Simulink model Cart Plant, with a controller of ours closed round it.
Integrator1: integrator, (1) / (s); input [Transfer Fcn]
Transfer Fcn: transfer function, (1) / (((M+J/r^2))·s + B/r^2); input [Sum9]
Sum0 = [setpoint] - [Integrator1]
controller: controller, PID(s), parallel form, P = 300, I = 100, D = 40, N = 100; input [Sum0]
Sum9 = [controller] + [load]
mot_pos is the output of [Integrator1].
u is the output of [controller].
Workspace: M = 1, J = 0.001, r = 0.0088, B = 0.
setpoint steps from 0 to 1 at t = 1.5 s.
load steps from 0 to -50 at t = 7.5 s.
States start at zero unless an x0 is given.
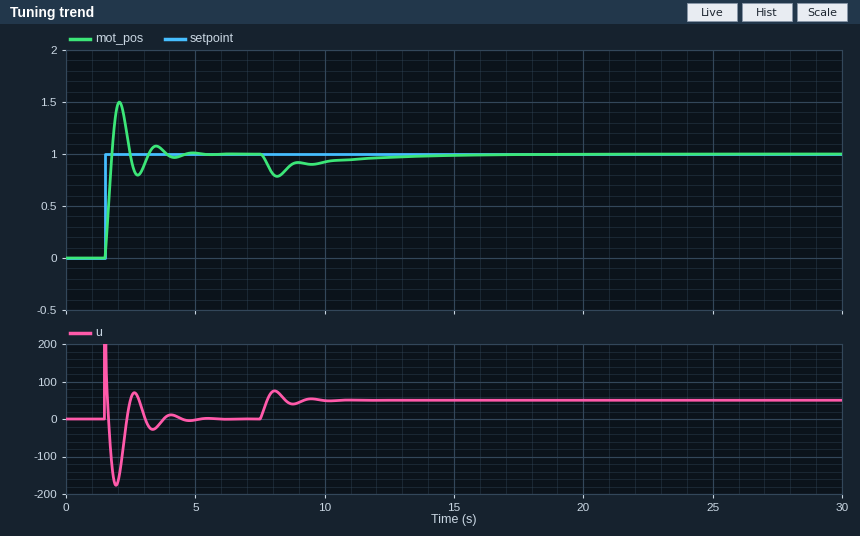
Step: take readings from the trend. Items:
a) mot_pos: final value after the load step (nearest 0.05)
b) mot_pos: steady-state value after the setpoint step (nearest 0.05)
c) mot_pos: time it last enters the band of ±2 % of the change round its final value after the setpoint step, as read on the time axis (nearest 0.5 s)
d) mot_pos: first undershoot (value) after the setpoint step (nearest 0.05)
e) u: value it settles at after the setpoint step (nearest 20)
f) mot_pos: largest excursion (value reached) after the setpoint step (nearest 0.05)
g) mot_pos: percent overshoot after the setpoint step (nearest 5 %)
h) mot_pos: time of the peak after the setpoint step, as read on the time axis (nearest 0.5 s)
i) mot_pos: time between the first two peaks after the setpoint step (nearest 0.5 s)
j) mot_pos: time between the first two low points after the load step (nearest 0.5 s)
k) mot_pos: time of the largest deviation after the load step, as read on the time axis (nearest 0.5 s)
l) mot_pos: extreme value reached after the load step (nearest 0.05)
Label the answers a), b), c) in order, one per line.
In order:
a) 1.00
b) 1.00
c) 4.5 s
d) 0.80
e) 0
f) 1.50
g) 50 %
h) 2.0 s
i) 1.5 s
j) 1.5 s
k) 8.0 s
l) 0.80
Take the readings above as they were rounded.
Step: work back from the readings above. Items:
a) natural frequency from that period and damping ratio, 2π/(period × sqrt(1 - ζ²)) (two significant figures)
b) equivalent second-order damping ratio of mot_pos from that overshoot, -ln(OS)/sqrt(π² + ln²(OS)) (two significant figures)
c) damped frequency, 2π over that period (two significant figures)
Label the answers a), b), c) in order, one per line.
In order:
a) 4.3 rad/s
b) 0.22
c) 4.2 rad/s
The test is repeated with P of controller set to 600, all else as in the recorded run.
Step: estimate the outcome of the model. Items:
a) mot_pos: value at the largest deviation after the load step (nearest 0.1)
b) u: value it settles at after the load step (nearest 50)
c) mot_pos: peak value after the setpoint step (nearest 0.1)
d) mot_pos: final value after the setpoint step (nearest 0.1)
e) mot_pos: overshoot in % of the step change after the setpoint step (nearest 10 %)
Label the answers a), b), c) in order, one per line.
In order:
a) 0.9
b) 50
c) 1.6
d) 1.0
e) 60 %
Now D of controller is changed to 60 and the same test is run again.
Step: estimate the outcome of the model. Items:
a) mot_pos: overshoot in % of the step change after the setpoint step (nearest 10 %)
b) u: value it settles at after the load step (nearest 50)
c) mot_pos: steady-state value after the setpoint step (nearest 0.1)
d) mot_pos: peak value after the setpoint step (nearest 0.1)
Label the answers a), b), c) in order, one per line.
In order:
a) 40 %
b) 50
c) 1.0
d) 1.4
